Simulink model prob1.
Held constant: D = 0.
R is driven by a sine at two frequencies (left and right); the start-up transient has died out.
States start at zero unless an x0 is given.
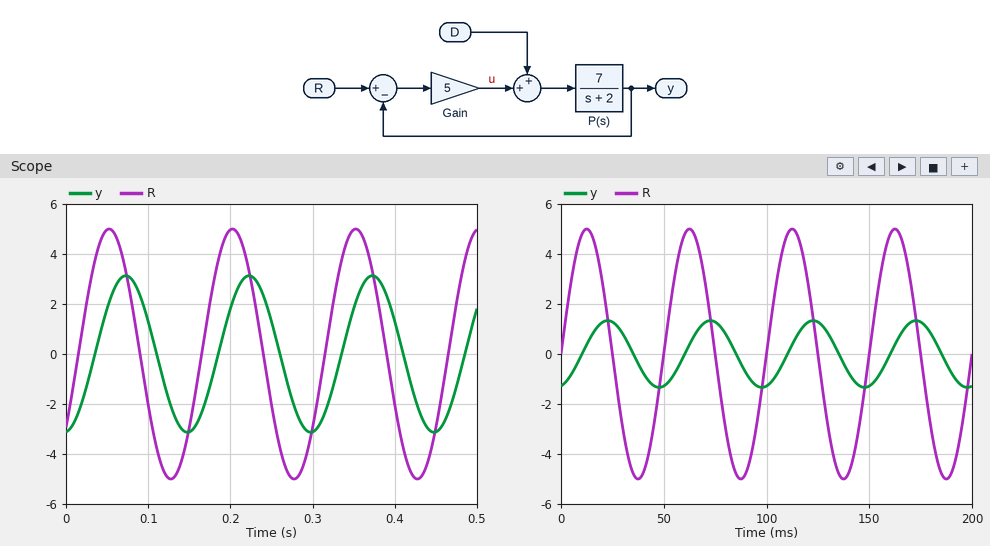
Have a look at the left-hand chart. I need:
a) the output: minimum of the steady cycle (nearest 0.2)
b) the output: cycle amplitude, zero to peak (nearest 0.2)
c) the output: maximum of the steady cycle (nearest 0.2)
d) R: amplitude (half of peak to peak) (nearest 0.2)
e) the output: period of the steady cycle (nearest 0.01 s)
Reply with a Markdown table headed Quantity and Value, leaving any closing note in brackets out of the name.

| Quantity | Value |
|---|---|
| the output: minimum of the steady cycle | -3.2 |
| the output: cycle amplitude, zero to peak | 3.2 |
| the output: maximum of the steady cycle | 3.2 |
| R: amplitude (half of peak to peak) | 5.0 |
| the output: period of the steady cycle | 0.15 s |
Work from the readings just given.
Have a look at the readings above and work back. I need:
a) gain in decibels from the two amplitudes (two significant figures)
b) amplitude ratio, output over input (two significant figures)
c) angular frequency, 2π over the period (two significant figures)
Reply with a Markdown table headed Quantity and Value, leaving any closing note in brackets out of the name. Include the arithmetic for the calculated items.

| Quantity | Value |
|---|---|
| gain in decibels from the two amplitudes | 20 log10(3.2 / 5) = -3.9 dB |
| amplitude ratio, output over input | 3.2 / 5 = 0.64 |
| angular frequency, 2π over the period | 2π / 0.15 = 42 rad/s |
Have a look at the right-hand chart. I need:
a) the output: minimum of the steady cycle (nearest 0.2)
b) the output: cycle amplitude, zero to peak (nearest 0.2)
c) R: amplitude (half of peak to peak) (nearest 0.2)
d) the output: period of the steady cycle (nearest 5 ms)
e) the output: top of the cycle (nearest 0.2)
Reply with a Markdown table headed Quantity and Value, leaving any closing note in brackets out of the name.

| Quantity | Value |
|---|---|
| the output: minimum of the steady cycle | -1.4 |
| the output: cycle amplitude, zero to peak | 1.4 |
| R: amplitude (half of peak to peak) | 5.0 |
| the output: period of the steady cycle | 50 ms |
| the output: top of the cycle | 1.4 |
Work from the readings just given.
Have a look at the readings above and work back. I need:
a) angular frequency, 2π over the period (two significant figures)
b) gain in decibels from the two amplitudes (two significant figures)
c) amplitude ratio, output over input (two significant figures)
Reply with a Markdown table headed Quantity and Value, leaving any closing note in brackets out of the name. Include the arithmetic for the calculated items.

| Quantity | Value |
|---|---|
| angular frequency, 2π over the period | 2π / 50 = 0.13 rad/ms |
| gain in decibels from the two amplitudes | 20 log10(1.4 / 5) = -11 dB |
| amplitude ratio, output over input | 1.4 / 5 = 0.28 |
